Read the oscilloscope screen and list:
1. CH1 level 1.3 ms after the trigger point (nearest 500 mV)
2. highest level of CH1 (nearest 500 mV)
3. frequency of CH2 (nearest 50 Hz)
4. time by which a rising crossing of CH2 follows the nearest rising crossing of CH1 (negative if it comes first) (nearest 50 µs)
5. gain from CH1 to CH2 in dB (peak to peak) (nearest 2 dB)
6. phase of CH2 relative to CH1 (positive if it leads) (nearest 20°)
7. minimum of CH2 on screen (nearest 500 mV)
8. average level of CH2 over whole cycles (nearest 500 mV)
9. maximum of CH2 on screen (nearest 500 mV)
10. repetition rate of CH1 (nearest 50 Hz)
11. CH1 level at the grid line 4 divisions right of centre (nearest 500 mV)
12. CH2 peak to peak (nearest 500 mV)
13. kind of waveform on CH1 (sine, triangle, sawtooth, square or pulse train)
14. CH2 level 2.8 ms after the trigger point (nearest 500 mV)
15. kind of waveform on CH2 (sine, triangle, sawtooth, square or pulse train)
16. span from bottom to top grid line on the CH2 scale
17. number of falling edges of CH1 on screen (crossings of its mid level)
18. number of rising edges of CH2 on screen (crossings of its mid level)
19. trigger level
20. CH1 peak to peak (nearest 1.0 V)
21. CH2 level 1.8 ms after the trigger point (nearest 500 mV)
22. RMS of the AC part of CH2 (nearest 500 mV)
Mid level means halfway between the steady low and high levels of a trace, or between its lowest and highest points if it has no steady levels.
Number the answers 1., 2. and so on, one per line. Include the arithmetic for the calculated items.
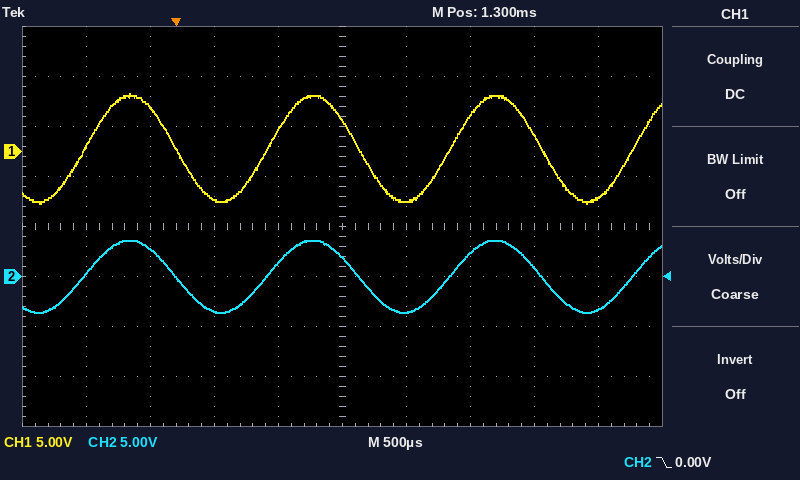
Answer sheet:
1. 3.0 V
2. 6.0 V
3. 700 Hz
4. 0 µs
5. 20 log10(7.0 V / 11.0 V) ≈ -4 dB
6. 0°
7. -3.5 V
8. (3.5 V + (-3.5 V)) / 2 ≈ 0.0 V
9. 3.5 V
10. 700 Hz
11. -4.5 V
12. 3.5 V − (-3.5 V) = 7.0 V
13. sine
14. 1.0 V
15. sine
16. 40 V
17. 3
18. 4
19. 0.00 V
20. 11.0 V
21. -3.5 V
22. 7.0 V / (2√2) ≈ 2.5 V
